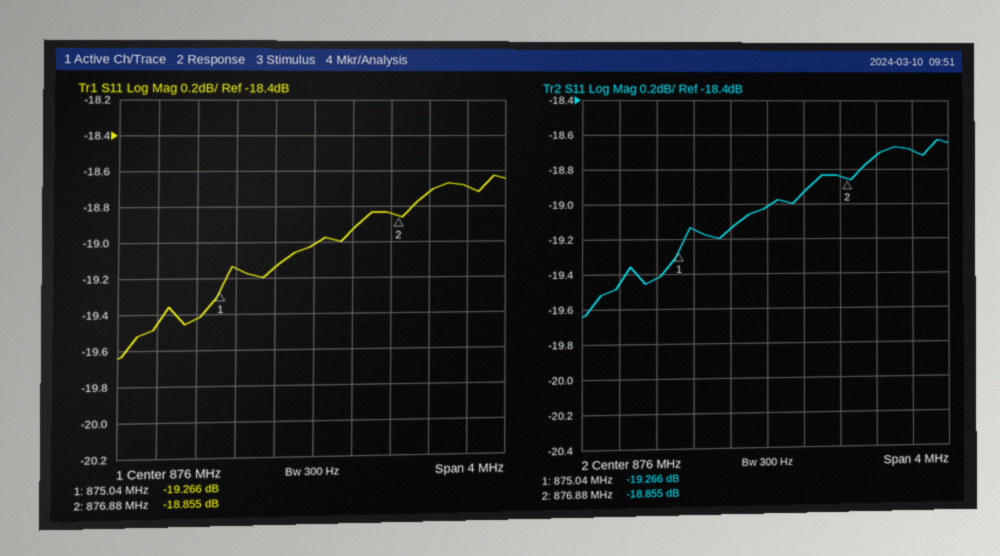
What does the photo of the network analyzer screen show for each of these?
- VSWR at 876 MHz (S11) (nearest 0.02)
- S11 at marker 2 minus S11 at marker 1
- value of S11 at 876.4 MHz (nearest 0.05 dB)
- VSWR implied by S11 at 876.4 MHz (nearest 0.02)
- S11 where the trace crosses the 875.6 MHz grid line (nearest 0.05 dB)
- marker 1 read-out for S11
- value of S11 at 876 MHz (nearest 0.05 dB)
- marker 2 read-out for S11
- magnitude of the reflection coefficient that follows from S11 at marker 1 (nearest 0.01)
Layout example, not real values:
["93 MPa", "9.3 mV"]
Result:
["1.26", "0.411 dB", "-18.95 dB", "1.26", "-19.15 dB", "-19.266 dB", "-19.00 dB", "-18.855 dB", "0.11"]
